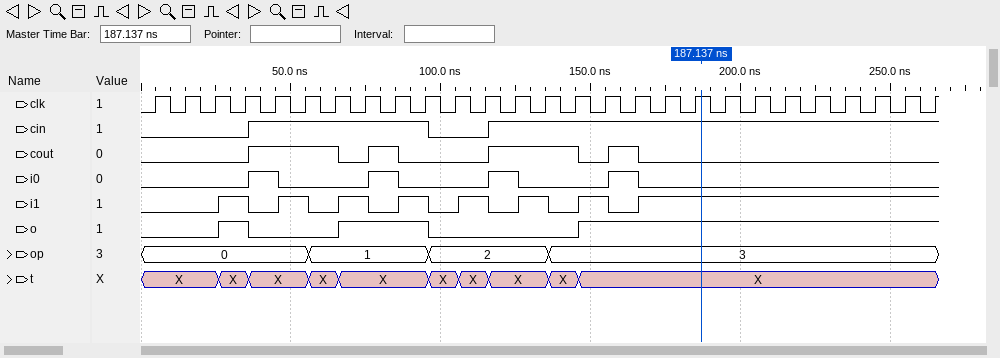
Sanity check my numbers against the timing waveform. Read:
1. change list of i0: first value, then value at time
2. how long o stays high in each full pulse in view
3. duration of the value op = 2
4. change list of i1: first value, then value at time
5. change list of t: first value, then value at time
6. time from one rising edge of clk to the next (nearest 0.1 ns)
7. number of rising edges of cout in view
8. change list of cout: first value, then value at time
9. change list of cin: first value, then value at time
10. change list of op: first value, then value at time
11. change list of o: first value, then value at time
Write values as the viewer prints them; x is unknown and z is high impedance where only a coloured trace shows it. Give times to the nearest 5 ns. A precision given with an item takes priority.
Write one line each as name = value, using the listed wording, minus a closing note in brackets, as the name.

change list of i0: first value, then value at time = 0, 1 at 35 ns, 0 at 45 ns, 1 at 75 ns, 0 at 85 ns, 1 at 115 ns, 0 at 125 ns, 1 at 155 ns, 0 at 165 ns
how long o stays high in each full pulse in view = 10 ns, 30 ns
duration of the value op = 2 = 40 ns
change list of i1: first value, then value at time = 0, 1 at 25 ns, 0 at 35 ns, 1 at 45 ns, 0 at 55 ns, 1 at 65 ns, 0 at 75 ns, 1 at 85 ns, 0 at 95 ns, 1 at 105 ns, 0 at 115 ns, 1 at 125 ns, 0 at 135 ns, 1 at 145 ns, 0 at 155 ns, 1 at 165 ns
change list of t: first value, then value at time = X, X at 25 ns, X at 35 ns, X at 55 ns, X at 65 ns, X at 95 ns, X at 105 ns, X at 115 ns, X at 135 ns, X at 145 ns
time from one rising edge of clk to the next = 10 ns
number of rising edges of cout in view = 4
change list of cout: first value, then value at time = 0, 1 at 35 ns, 0 at 65 ns, 1 at 75 ns, 0 at 85 ns, 1 at 115 ns, 0 at 145 ns, 1 at 155 ns, 0 at 165 ns
change list of cin: first value, then value at time = 0, 1 at 35 ns, 0 at 95 ns, 1 at 115 ns
change list of op: first value, then value at time = 0, 1 at 55 ns, 2 at 95 ns, 3 at 135 ns
change list of o: first value, then value at time = 0, 1 at 25 ns, 0 at 35 ns, 1 at 65 ns, 0 at 95 ns, 1 at 145 ns
